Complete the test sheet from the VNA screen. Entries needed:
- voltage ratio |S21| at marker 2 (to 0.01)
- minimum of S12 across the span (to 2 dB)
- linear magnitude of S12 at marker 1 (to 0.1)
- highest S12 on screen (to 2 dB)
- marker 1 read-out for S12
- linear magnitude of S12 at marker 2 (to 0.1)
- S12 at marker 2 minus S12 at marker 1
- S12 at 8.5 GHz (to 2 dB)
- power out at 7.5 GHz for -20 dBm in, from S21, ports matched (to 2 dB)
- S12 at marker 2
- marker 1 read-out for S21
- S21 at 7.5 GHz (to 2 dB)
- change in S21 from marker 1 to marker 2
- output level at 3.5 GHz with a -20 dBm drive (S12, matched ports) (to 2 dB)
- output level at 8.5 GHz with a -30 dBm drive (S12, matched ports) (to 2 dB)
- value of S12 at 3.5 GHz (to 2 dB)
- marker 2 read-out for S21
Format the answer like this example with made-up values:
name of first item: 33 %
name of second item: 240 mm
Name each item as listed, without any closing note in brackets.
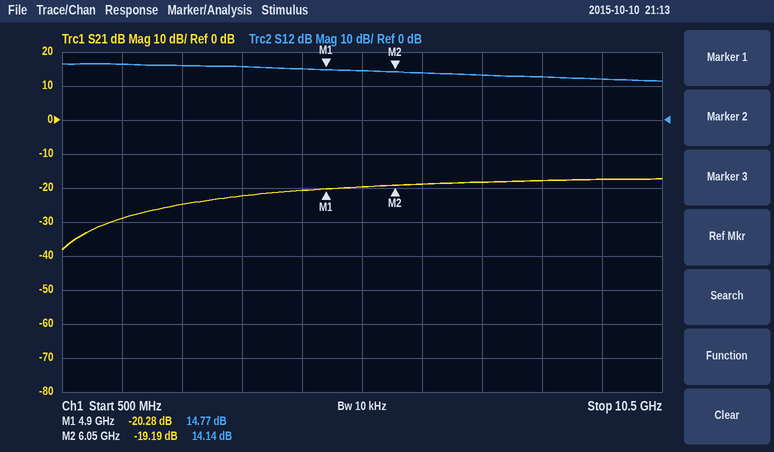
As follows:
voltage ratio |S21| at marker 2: 0.11
minimum of S12 across the span: 12 dB
linear magnitude of S12 at marker 1: 5.5
highest S12 on screen: 16 dB
marker 1 read-out for S12: 14.77 dB
linear magnitude of S12 at marker 2: 5.1
S12 at marker 2 minus S12 at marker 1: -0.63 dB
S12 at 8.5 GHz: 12 dB
power out at 7.5 GHz for -20 dBm in, from S21, ports matched: -38 dBm
S12 at marker 2: 14.14 dB
marker 1 read-out for S21: -20.28 dB
S21 at 7.5 GHz: -18 dB
change in S21 from marker 1 to marker 2: 1.09 dB
output level at 3.5 GHz with a -20 dBm drive (S12, matched ports): -4 dBm
output level at 8.5 GHz with a -30 dBm drive (S12, matched ports): -18 dBm
value of S12 at 3.5 GHz: 16 dB
marker 2 read-out for S21: -19.19 dB
